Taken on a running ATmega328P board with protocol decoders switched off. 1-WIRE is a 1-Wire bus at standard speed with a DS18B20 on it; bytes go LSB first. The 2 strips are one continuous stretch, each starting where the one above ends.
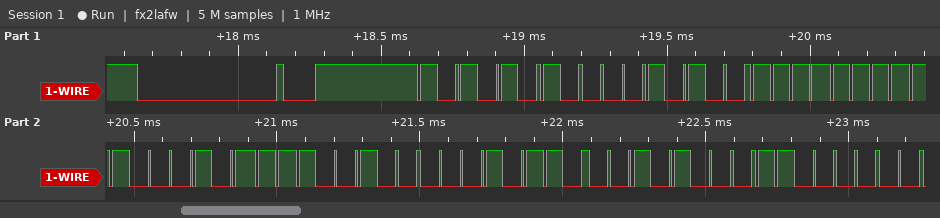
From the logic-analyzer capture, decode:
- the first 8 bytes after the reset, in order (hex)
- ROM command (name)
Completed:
55 28 FF A3 27 68 14 03
Match ROM
